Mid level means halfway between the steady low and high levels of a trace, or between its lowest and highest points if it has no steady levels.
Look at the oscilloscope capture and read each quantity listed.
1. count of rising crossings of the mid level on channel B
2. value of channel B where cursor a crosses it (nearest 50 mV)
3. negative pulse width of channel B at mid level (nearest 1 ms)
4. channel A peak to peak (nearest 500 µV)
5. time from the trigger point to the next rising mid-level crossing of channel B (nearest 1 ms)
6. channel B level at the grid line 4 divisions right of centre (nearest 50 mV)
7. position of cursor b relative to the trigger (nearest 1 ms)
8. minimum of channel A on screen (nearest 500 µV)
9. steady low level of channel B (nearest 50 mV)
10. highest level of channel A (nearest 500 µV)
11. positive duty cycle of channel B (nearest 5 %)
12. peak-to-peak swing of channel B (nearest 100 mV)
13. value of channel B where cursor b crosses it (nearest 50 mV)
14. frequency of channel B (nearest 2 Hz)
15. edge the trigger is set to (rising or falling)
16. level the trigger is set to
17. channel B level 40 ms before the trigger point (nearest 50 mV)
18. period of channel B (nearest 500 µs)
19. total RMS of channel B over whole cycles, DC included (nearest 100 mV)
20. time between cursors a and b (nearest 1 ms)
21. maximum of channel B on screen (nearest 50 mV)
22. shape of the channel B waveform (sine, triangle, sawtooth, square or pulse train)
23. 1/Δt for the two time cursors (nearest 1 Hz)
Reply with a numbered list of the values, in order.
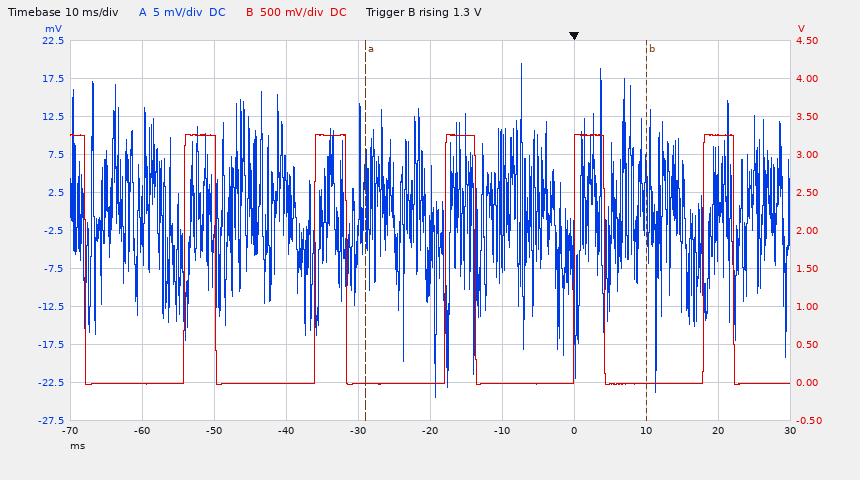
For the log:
1. 5
2. 0 mV
3. 14 ms
4. 44.0 mV
5. 18 ms
6. 3.25 V
7. +10 ms
8. -24.5 mV
9. 0 mV
10. 19.5 mV
11. 25 %
12. 3.30 V
13. 0 mV
14. 56 Hz
15. rising
16. 1.3 V
17. 0 mV
18. 18.0 ms
19. 1.6 V
20. 39 ms
21. 3.25 V
22. pulse train
23. 26 Hz
